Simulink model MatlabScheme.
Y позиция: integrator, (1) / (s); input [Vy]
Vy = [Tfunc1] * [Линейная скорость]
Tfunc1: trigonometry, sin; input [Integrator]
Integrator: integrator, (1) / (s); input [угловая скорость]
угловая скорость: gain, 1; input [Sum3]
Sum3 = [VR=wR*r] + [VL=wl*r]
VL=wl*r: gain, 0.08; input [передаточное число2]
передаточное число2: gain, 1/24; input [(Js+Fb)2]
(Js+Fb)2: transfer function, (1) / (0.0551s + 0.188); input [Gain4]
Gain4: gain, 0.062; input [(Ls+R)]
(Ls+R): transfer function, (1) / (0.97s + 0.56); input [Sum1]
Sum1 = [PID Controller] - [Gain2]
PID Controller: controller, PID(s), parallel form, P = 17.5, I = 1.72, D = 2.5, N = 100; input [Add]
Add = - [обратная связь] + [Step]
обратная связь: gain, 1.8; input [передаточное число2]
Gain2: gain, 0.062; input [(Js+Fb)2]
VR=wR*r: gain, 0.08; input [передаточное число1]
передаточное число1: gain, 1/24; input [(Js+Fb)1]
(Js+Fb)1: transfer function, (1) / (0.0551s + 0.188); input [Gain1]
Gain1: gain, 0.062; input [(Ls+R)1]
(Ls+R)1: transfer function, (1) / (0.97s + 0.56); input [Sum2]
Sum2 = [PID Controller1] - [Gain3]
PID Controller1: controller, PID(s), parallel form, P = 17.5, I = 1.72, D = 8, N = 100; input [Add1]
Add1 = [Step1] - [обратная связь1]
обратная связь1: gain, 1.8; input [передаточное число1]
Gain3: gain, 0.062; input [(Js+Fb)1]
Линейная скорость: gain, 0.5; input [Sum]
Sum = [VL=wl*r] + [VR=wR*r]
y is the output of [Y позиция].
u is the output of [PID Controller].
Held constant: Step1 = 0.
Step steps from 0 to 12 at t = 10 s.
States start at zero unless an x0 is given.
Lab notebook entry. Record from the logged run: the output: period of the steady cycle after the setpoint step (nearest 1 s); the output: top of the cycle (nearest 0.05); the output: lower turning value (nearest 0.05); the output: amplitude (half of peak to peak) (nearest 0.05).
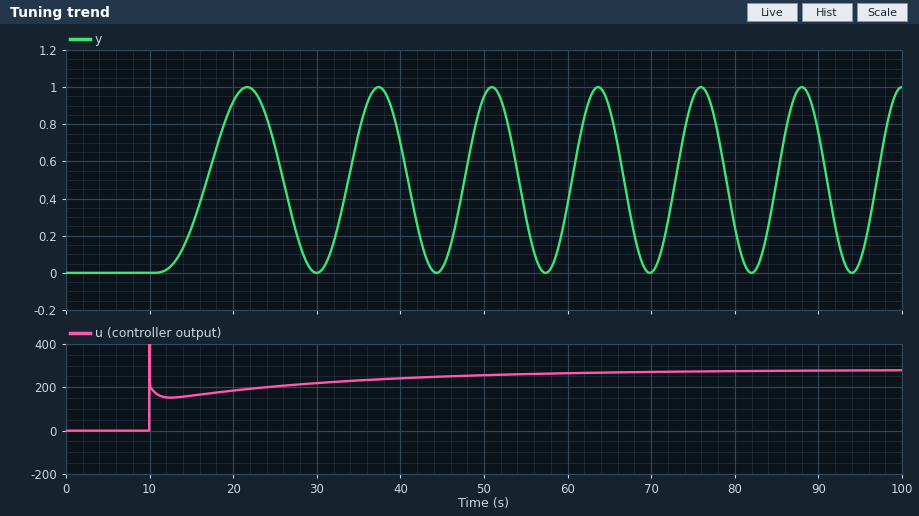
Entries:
12 s
1.00
0.00
0.50
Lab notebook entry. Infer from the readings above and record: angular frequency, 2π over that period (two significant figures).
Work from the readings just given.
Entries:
0.52 rad/s
